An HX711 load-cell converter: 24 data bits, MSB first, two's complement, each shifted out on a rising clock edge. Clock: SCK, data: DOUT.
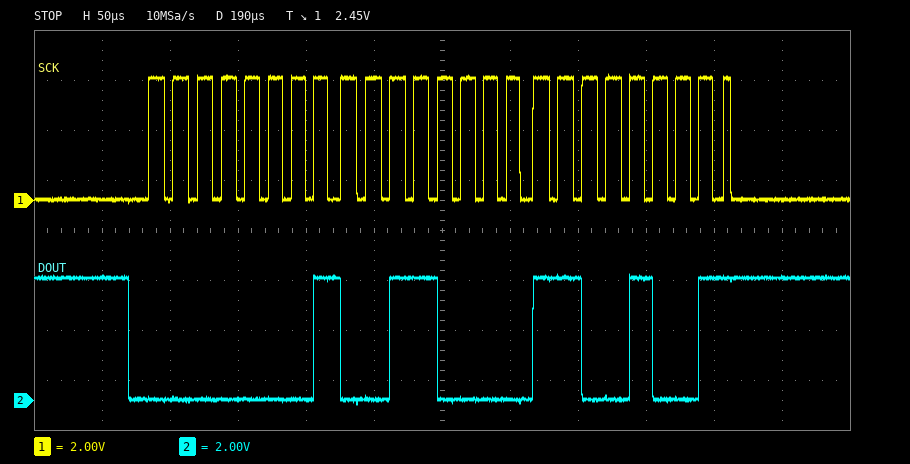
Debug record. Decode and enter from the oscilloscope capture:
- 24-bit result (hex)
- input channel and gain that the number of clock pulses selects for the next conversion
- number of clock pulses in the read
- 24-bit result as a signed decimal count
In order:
0x0130C9
channel A, gain 128
25
78025
